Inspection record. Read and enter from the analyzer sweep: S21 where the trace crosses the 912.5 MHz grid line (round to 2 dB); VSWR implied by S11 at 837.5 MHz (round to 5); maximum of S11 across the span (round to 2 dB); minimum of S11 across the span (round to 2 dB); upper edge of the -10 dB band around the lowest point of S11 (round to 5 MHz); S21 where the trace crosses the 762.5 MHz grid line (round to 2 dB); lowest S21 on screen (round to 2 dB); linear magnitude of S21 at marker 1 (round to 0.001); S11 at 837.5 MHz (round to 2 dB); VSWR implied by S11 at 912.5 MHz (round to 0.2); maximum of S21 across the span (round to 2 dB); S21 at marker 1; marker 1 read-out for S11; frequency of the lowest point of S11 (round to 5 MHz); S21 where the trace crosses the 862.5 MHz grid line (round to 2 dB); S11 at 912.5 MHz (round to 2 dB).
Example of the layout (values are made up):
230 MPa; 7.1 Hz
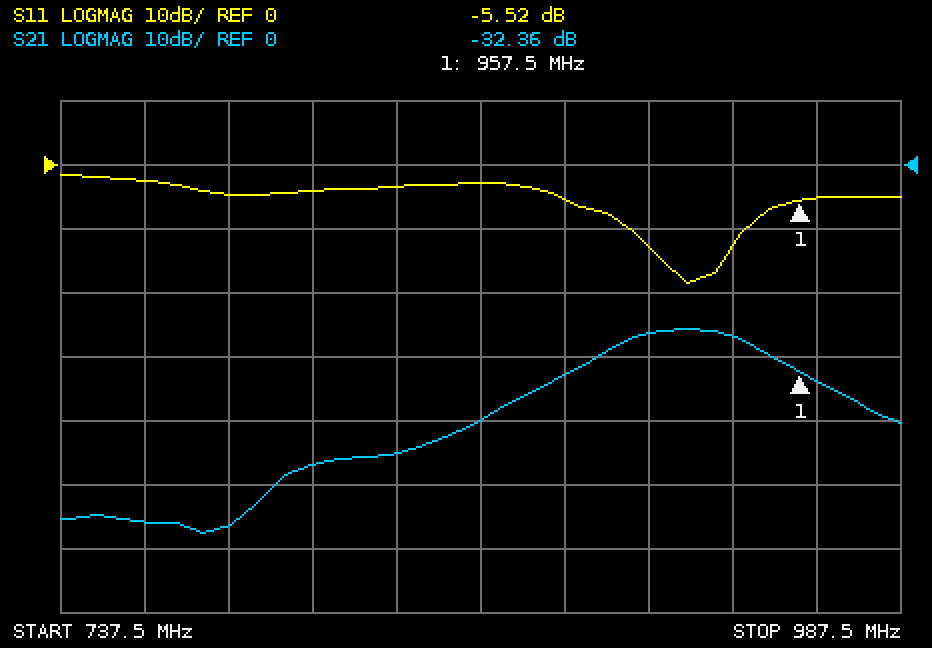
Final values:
-26 dB; 5; -2 dB; -18 dB; 940 MHz; -56 dB; -58 dB; 0.024; -4 dB; 1.6; -26 dB; -32.36 dB; -5.52 dB; 925 MHz; -40 dB; -12 dB
